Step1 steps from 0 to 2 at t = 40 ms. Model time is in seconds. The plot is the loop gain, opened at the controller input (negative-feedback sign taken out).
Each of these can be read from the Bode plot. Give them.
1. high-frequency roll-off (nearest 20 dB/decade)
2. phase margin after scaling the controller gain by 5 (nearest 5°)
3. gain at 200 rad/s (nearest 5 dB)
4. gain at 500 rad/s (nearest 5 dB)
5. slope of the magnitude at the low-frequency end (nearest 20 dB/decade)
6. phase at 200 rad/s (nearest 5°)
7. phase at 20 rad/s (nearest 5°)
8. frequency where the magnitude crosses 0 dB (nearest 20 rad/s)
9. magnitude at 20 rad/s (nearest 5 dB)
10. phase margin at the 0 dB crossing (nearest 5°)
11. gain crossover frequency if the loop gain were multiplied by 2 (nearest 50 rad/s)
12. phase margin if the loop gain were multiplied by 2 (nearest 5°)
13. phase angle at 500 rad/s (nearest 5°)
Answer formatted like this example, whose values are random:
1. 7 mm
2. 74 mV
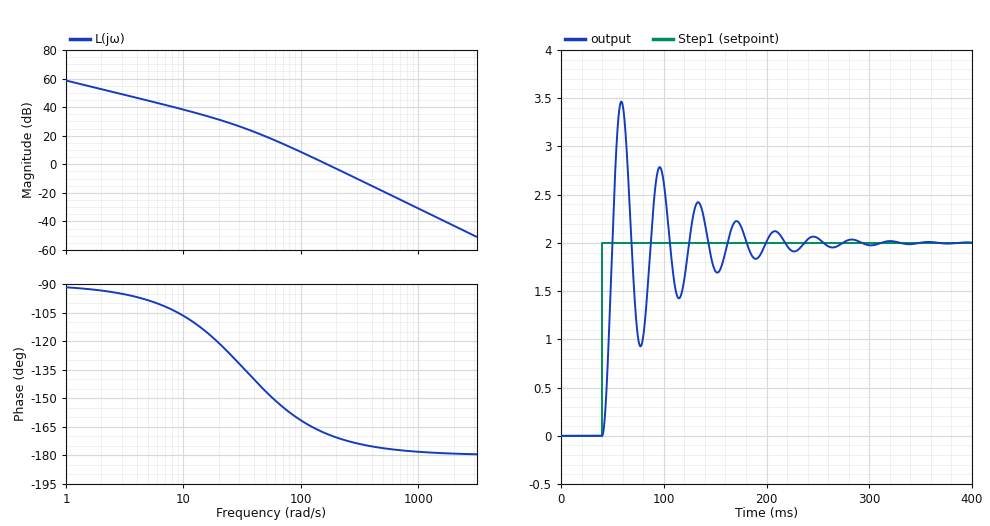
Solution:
1. -40 dB/decade
2. 5°
3. -5 dB
4. -20 dB
5. -20 dB/decade
6. -170°
7. -120°
8. 160 rad/s
9. 30 dB
10. 10°
11. 250 rad/s
12. 10°
13. -175°
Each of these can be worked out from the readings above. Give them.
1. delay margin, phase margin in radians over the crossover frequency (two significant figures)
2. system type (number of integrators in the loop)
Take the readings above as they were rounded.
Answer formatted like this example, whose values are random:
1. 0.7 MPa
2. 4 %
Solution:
1. 0.0011 s
2. 1
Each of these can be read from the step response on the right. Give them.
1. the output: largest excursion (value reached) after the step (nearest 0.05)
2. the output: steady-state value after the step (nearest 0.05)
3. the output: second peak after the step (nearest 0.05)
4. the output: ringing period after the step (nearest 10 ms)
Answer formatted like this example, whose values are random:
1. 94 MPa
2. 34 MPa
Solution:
1. 3.45
2. 2.00
3. 2.80
4. 40 ms
